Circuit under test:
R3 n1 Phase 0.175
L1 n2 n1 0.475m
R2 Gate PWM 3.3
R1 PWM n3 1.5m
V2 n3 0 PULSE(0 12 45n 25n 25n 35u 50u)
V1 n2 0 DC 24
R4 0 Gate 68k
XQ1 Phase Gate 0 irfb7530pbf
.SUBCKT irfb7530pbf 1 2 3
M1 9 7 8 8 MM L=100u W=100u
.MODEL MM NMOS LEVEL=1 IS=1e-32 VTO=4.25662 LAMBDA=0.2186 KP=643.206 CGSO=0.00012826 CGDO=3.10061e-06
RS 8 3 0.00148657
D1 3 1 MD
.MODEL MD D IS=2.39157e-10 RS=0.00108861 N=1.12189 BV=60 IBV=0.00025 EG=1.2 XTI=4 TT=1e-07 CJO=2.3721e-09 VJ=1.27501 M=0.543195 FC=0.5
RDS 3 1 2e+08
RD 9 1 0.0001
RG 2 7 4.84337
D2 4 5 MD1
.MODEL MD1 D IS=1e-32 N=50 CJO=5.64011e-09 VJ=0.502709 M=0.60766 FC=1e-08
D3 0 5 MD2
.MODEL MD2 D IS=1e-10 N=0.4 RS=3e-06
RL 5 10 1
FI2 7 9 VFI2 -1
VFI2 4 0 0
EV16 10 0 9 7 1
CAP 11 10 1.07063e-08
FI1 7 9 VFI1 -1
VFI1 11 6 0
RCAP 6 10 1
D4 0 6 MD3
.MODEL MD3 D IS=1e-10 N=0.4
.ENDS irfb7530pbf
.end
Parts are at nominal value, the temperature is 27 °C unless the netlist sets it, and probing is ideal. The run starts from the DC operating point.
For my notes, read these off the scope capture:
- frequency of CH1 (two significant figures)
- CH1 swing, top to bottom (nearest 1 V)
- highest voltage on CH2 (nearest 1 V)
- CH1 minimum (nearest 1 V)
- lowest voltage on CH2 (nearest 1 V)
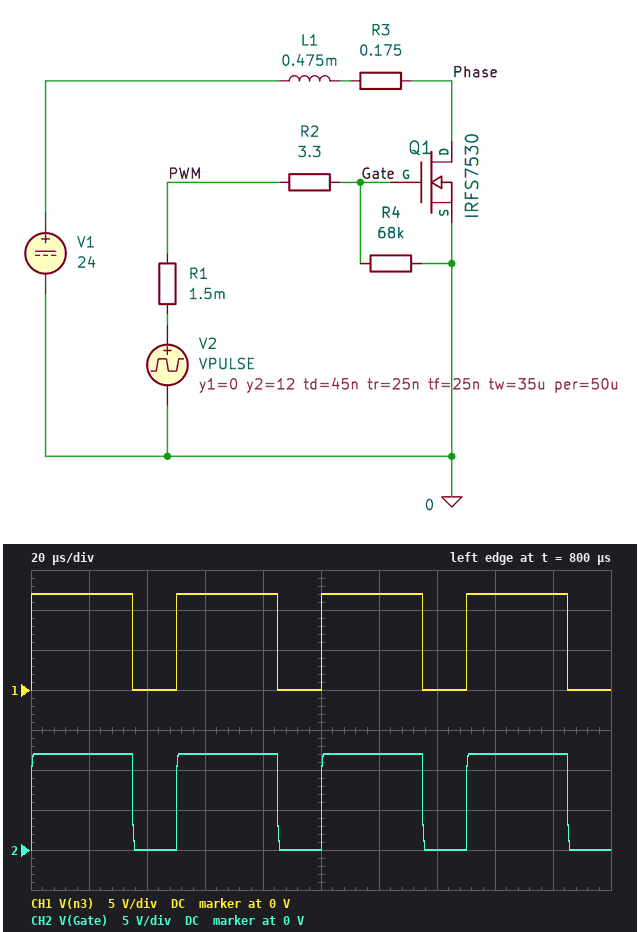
20 kHz
12 V
12 V
0 V
0 V
